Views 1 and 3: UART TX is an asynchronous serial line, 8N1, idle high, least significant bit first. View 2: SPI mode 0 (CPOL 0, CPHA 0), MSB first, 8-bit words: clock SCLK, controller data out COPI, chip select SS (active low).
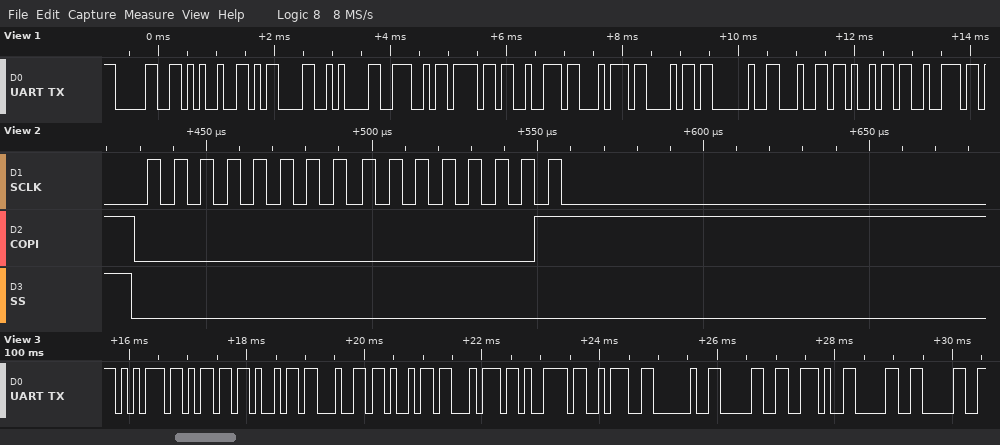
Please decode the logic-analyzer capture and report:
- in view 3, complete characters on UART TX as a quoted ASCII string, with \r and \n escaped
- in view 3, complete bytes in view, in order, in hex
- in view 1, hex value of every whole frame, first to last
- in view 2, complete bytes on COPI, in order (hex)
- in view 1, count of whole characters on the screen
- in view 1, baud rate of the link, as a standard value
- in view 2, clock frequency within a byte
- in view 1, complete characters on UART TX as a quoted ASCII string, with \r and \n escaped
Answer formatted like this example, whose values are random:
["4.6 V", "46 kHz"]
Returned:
["\"umidity: 0.00\"", "75 6D 69 64 69 74 79 3A 20 30 2E 30 30", "30 25 0D 0A 4E 6F 72 74 68 20 64 69 72", "00 01", "13", "9600 baud", "125 kHz", "\"0%\\r\\nNorth dir\""]
